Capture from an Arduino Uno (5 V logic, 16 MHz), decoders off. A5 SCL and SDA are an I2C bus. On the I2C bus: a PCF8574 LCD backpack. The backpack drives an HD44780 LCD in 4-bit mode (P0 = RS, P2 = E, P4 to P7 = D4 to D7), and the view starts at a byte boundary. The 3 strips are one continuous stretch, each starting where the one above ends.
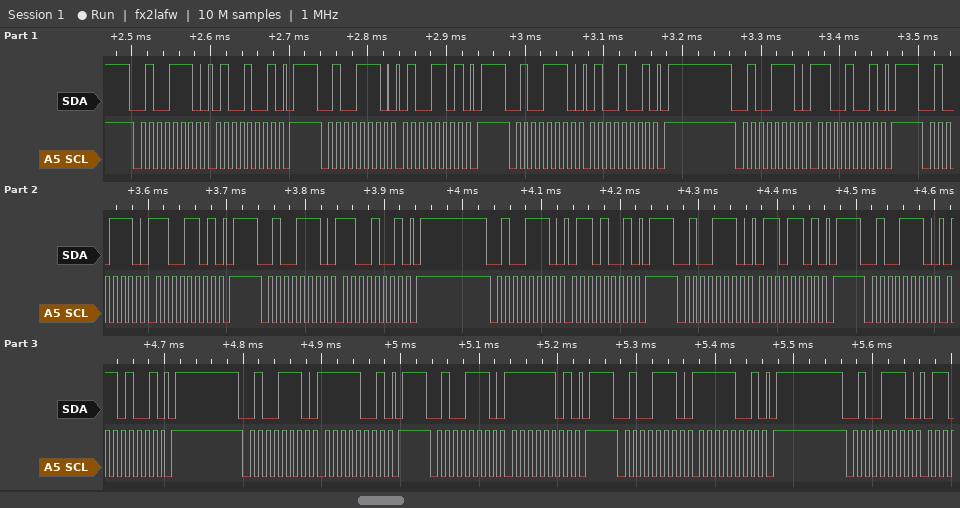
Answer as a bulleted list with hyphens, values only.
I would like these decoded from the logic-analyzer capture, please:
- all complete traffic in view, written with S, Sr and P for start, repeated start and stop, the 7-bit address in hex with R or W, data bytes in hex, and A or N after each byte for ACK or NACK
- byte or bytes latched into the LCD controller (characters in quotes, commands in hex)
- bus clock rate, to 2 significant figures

- S 27W A 49 A P S 27W A 4D A P S 27W A 49 A P S 27W A C9 A P S 27W A CD A P S 27W A C9 A P S 27W A 69 A P S 27W A 6D A P S 27W A 69 A P S 27W A F9 A P S 27W A FD A P S 27W A F9 A P S 27W A
- 'L' 'o'
- 100 kHz
